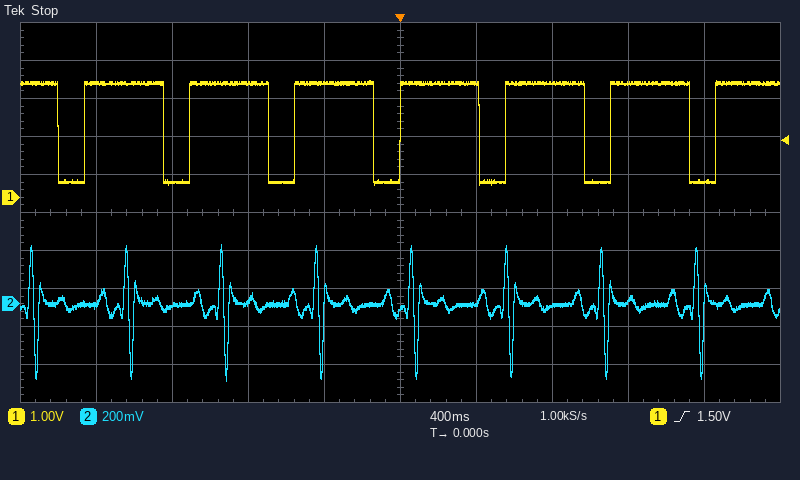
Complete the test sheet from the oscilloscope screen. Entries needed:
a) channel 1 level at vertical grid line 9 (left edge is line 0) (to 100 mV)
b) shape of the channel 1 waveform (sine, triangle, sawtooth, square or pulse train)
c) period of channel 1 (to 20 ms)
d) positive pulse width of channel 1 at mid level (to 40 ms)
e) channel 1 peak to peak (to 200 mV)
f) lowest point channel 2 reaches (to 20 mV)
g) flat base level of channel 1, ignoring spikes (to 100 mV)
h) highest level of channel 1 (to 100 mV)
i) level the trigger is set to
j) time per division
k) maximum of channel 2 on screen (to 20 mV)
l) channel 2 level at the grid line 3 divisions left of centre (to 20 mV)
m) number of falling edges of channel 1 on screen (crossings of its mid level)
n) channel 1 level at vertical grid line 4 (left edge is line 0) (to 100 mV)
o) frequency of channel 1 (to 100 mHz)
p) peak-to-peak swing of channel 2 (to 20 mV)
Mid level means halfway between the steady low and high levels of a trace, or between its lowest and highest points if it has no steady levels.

400 mV
pulse train
560 ms
400 ms
2.8 V
-400 mV
400 mV
3.1 V
1.50 V
400 ms
320 mV
0 mV
7
3.0 V
1.8 Hz
720 mV
